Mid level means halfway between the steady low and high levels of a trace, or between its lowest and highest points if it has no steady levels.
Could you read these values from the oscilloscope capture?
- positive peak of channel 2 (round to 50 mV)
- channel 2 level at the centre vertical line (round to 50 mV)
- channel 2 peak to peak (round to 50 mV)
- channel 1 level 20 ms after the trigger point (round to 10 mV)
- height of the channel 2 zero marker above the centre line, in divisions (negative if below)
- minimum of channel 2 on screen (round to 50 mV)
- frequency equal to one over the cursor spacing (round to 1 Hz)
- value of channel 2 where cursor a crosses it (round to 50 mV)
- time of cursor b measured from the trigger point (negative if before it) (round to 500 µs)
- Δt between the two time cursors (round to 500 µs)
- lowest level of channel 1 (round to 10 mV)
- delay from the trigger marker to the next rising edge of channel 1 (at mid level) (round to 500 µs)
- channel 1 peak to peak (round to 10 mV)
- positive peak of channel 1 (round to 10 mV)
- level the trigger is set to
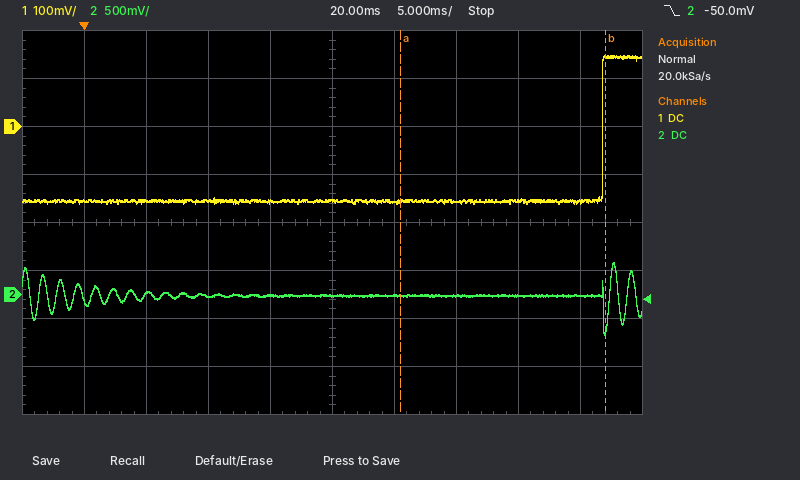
350 mV
0 mV
750 mV
-150 mV
-1.5 div
-400 mV
61 Hz
0 mV
+42.0 ms
16.5 ms
-160 mV
42.0 ms
310 mV
150 mV
-50.0 mV
